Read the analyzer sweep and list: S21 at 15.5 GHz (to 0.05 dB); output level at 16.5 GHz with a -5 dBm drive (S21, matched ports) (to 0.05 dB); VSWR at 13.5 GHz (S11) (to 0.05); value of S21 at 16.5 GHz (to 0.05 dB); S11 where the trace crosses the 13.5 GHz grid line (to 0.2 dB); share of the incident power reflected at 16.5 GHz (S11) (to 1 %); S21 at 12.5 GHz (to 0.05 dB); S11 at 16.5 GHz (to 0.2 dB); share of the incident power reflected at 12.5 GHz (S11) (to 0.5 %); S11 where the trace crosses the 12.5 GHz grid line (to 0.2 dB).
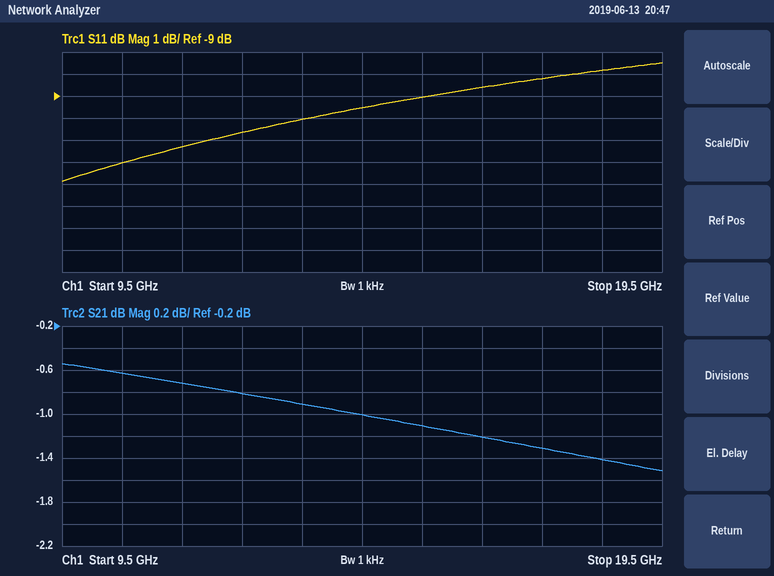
-1.10 dB
-6.20 dBm
1.90
-1.20 dB
-10.0 dB
14 %
-0.80 dB
-8.6 dB
8.5 %
-10.6 dB
